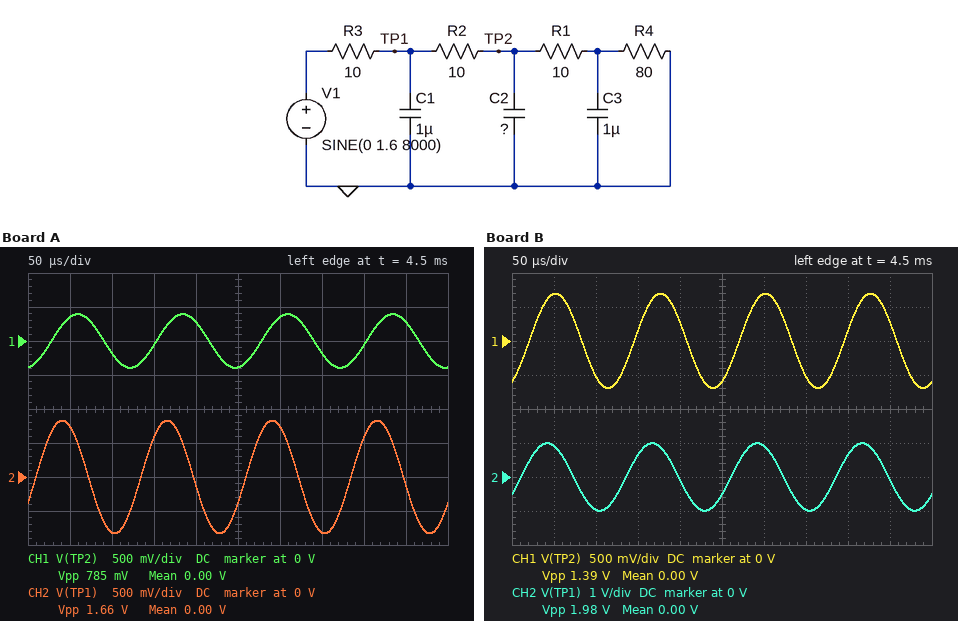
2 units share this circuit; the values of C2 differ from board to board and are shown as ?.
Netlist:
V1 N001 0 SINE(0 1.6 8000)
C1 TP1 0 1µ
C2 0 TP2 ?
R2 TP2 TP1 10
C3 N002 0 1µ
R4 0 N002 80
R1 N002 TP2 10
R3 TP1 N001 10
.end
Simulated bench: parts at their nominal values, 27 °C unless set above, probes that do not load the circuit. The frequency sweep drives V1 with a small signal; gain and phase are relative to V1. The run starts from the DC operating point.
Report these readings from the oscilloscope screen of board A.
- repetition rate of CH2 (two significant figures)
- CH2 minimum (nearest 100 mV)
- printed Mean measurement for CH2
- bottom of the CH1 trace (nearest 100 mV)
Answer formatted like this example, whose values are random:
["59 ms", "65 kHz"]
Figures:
["8.0 kHz", "-800 mV", "0.00 V", "-400 mV"]
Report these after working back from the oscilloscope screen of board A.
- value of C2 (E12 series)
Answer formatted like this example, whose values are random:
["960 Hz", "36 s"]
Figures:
["2.7 µF"]
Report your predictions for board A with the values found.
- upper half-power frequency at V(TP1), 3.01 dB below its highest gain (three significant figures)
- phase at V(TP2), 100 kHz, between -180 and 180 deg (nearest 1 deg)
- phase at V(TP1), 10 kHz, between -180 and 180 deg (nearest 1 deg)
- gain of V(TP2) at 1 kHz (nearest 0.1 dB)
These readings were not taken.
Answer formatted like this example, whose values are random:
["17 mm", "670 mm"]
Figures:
["3.71 kHz", "-156 deg", "-29 deg", "-2.4 dB"]
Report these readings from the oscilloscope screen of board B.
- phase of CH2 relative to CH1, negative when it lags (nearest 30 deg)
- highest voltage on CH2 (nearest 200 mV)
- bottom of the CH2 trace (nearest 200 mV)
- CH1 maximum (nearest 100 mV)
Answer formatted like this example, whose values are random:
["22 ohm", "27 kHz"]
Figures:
["30 deg", "1.0 V", "-1.0 V", "700 mV"]
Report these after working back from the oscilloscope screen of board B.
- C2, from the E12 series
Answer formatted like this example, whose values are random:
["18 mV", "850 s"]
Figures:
["680 nF"]
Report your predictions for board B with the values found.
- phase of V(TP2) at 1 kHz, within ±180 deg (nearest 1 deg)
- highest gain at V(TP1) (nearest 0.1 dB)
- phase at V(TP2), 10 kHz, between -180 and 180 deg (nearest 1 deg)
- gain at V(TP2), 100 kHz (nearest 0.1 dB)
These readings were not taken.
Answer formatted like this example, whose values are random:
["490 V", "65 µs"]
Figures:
["-12 deg", "-0.8 dB", "-65 deg", "-30.3 dB"]
